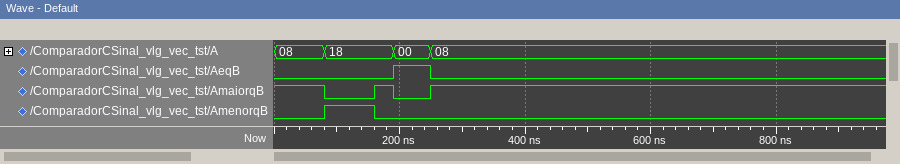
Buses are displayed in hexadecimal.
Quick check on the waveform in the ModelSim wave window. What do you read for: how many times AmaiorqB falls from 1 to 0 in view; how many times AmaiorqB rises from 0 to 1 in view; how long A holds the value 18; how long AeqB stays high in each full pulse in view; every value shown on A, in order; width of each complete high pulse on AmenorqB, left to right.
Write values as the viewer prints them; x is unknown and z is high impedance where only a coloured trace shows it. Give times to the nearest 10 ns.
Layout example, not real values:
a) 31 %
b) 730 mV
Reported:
a) 2
b) 2
c) 110 ns
d) 60 ns
e) 08, 18, 00, 08
f) 80 ns
